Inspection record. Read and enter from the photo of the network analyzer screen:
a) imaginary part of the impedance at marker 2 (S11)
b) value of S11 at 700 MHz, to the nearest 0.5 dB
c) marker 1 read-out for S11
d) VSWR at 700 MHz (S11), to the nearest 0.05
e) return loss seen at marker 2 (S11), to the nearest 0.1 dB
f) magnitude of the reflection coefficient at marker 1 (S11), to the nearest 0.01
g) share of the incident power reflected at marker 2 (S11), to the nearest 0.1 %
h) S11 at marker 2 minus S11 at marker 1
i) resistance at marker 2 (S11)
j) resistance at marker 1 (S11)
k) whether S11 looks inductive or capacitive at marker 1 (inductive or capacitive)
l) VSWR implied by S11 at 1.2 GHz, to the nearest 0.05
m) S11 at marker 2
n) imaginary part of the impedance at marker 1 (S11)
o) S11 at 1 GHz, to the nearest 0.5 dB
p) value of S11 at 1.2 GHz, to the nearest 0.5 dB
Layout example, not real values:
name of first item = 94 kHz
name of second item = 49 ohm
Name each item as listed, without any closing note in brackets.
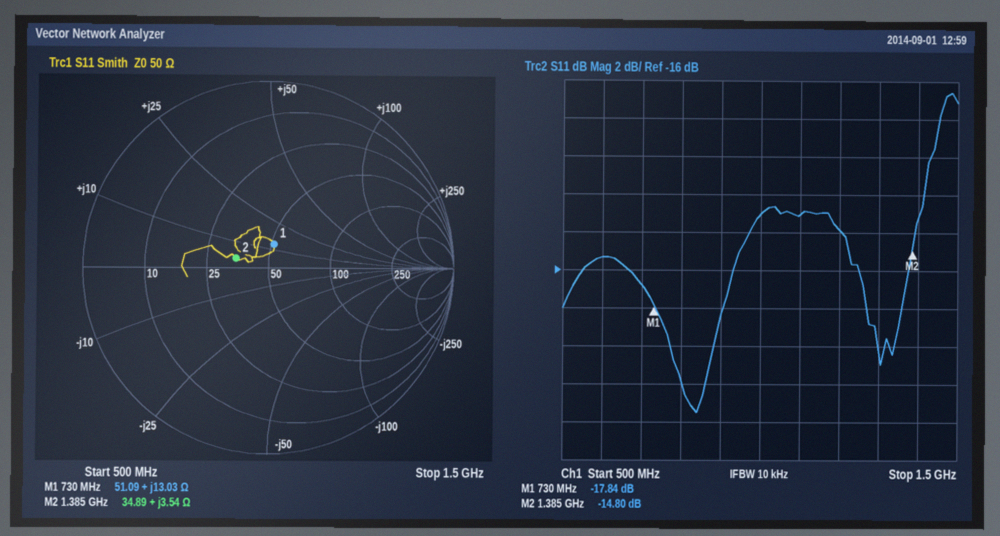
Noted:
imaginary part of the impedance at marker 2 = +3.54 Ω
value of S11 at 700 MHz, to the nearest 0.5 dB = -17.0 dB
marker 1 read-out for S11 = -17.84 dB
VSWR at 700 MHz (S11), to the nearest 0.05 = 1.35
return loss seen at marker 2 (S11), to the nearest 0.1 dB = 14.8 dB
magnitude of the reflection coefficient at marker 1 (S11), to the nearest 0.01 = 0.13
share of the incident power reflected at marker 2 (S11), to the nearest 0.1 % = 3.3 %
S11 at marker 2 minus S11 at marker 1 = 3.04 dB
resistance at marker 2 = 34.89 Ω
resistance at marker 1 = 51.09 Ω
whether S11 looks inductive or capacitive at marker 1 = inductive
VSWR implied by S11 at 1.2 GHz, to the nearest 0.05 = 1.50
S11 at marker 2 = -14.80 dB
imaginary part of the impedance at marker 1 = +13.03 Ω
S11 at 1 GHz, to the nearest 0.5 dB = -13.0 dB
value of S11 at 1.2 GHz, to the nearest 0.5 dB = -14.0 dB
